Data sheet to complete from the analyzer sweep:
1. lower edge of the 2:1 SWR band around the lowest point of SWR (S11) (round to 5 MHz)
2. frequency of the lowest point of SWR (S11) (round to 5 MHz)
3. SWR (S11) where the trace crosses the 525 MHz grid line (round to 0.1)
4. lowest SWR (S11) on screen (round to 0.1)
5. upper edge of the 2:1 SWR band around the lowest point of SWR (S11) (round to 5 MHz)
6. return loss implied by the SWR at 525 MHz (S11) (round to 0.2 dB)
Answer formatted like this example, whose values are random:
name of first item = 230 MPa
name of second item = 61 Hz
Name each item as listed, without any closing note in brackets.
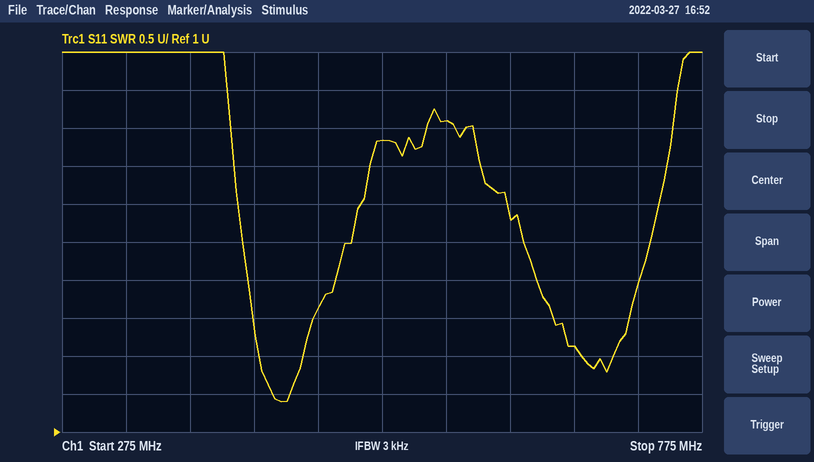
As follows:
lower edge of the 2:1 SWR band around the lowest point of SWR (S11) = 430 MHz
frequency of the lowest point of SWR (S11) = 445 MHz
SWR (S11) where the trace crosses the 525 MHz grid line = 4.8
lowest SWR (S11) on screen = 1.4
upper edge of the 2:1 SWR band around the lowest point of SWR (S11) = 465 MHz
return loss implied by the SWR at 525 MHz (S11) = 3.6 dB
